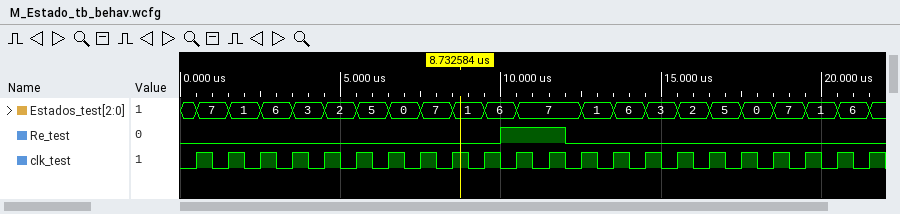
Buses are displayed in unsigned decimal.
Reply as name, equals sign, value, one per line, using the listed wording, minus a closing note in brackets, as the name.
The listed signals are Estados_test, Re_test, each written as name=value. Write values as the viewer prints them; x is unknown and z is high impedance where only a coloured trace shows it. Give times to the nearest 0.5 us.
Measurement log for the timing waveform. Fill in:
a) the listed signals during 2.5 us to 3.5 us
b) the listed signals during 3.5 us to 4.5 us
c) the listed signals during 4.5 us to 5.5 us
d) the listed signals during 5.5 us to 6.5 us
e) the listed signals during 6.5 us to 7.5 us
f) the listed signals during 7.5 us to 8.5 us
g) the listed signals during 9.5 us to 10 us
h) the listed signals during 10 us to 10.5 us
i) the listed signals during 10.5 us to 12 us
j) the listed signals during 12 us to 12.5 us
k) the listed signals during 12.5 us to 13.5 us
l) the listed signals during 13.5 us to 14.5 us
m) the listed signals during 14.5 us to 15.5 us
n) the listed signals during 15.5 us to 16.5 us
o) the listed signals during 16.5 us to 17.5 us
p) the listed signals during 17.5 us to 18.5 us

the listed signals during 2.5 us to 3.5 us = Estados_test=6, Re_test=0
the listed signals during 3.5 us to 4.5 us = Estados_test=3, Re_test=0
the listed signals during 4.5 us to 5.5 us = Estados_test=2, Re_test=0
the listed signals during 5.5 us to 6.5 us = Estados_test=5, Re_test=0
the listed signals during 6.5 us to 7.5 us = Estados_test=0, Re_test=0
the listed signals during 7.5 us to 8.5 us = Estados_test=7, Re_test=0
the listed signals during 9.5 us to 10 us = Estados_test=6, Re_test=0
the listed signals during 10 us to 10.5 us = Estados_test=6, Re_test=1
the listed signals during 10.5 us to 12 us = Estados_test=7, Re_test=1
the listed signals during 12 us to 12.5 us = Estados_test=7, Re_test=0
the listed signals during 12.5 us to 13.5 us = Estados_test=1, Re_test=0
the listed signals during 13.5 us to 14.5 us = Estados_test=6, Re_test=0
the listed signals during 14.5 us to 15.5 us = Estados_test=3, Re_test=0
the listed signals during 15.5 us to 16.5 us = Estados_test=2, Re_test=0
the listed signals during 16.5 us to 17.5 us = Estados_test=5, Re_test=0
the listed signals during 17.5 us to 18.5 us = Estados_test=0, Re_test=0
